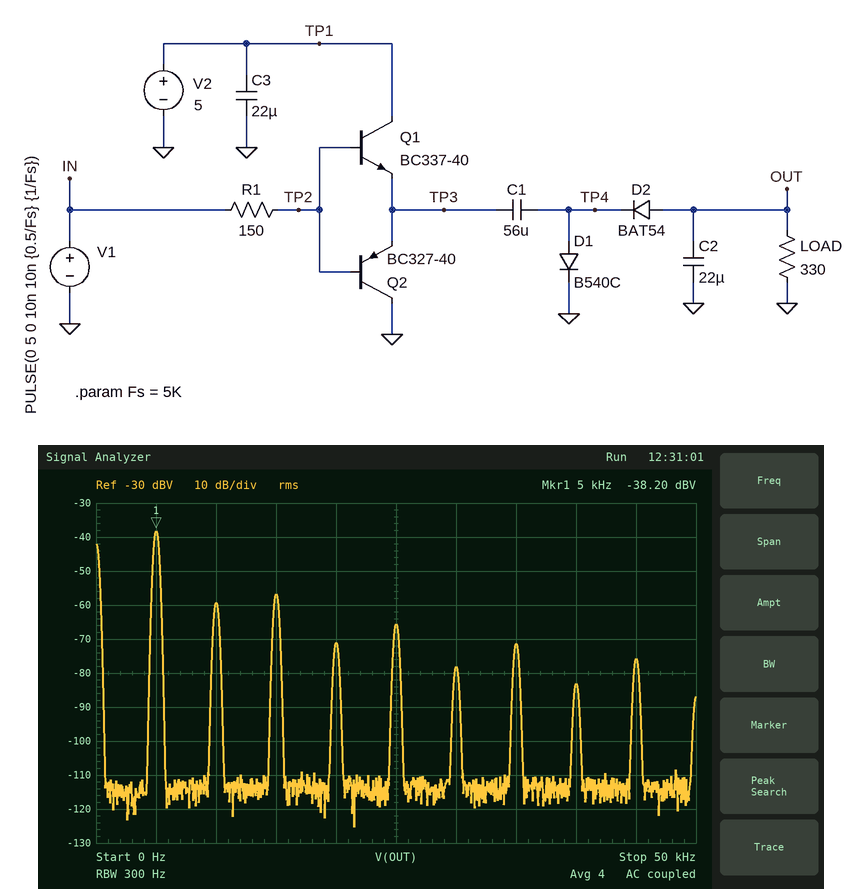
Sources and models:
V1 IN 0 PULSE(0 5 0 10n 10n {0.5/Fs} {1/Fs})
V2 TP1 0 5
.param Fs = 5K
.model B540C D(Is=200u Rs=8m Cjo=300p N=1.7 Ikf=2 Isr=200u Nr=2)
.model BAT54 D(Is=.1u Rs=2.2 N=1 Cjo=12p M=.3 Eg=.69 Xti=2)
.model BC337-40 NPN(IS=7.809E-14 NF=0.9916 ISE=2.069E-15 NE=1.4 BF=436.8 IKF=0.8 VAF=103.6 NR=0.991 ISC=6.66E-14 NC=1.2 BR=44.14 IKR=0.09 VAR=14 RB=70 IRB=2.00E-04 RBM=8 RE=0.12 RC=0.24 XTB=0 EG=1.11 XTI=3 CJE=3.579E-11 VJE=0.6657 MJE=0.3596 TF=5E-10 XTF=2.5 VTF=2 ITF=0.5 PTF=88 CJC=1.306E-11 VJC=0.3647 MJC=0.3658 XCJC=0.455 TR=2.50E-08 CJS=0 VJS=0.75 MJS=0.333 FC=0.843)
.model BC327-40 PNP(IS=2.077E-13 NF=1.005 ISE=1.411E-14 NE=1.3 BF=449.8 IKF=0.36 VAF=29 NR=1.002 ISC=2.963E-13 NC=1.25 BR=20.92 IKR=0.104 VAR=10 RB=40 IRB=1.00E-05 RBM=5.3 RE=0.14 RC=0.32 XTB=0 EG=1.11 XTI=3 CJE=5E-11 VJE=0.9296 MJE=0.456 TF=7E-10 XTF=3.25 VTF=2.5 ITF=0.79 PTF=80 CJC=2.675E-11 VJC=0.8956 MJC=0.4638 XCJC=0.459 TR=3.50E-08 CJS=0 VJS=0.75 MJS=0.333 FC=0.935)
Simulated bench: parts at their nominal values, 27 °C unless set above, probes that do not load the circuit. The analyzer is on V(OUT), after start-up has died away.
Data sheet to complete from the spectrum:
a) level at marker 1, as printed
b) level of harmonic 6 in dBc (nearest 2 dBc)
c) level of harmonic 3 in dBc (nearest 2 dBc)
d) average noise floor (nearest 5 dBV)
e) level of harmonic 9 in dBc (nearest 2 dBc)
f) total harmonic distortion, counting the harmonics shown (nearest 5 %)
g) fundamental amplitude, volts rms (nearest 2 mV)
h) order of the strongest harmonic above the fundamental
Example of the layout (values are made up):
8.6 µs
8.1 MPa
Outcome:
-38.20 dBV
-40 dBc
-18 dBc
-115 dBV
-38 dBc
15 %
12 mV
3
